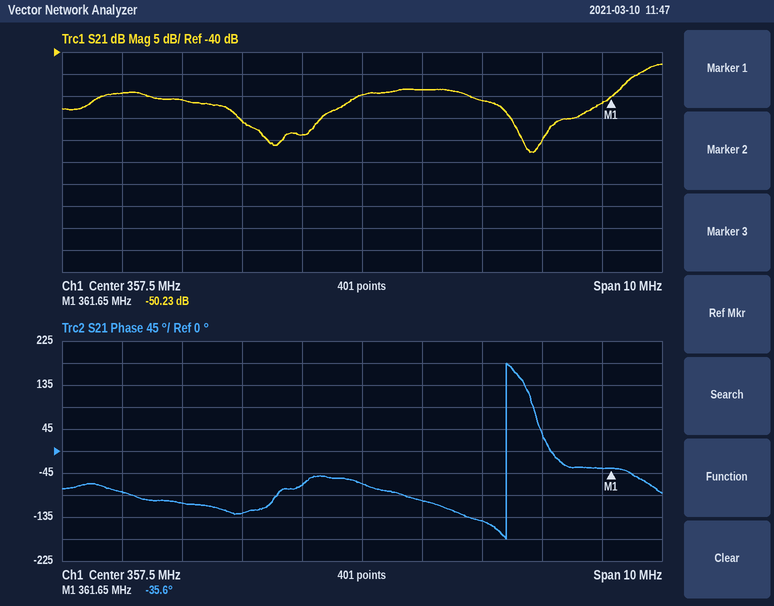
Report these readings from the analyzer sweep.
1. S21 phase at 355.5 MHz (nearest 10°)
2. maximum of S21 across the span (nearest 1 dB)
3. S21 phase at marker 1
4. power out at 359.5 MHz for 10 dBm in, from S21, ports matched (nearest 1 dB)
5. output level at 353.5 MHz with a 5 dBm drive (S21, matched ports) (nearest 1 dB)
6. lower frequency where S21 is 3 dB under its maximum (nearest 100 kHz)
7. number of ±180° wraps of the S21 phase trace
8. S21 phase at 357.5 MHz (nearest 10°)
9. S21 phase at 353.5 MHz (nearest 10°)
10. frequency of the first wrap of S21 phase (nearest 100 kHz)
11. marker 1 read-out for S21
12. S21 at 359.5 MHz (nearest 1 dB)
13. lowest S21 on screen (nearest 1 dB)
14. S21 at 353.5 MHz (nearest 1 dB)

-130°
-43 dB
-35.6°
-41 dBm
-44 dBm
362.0 MHz
1
-70°
-80°
359.9 MHz
-50.23 dB
-51 dB
-63 dB
-49 dB
